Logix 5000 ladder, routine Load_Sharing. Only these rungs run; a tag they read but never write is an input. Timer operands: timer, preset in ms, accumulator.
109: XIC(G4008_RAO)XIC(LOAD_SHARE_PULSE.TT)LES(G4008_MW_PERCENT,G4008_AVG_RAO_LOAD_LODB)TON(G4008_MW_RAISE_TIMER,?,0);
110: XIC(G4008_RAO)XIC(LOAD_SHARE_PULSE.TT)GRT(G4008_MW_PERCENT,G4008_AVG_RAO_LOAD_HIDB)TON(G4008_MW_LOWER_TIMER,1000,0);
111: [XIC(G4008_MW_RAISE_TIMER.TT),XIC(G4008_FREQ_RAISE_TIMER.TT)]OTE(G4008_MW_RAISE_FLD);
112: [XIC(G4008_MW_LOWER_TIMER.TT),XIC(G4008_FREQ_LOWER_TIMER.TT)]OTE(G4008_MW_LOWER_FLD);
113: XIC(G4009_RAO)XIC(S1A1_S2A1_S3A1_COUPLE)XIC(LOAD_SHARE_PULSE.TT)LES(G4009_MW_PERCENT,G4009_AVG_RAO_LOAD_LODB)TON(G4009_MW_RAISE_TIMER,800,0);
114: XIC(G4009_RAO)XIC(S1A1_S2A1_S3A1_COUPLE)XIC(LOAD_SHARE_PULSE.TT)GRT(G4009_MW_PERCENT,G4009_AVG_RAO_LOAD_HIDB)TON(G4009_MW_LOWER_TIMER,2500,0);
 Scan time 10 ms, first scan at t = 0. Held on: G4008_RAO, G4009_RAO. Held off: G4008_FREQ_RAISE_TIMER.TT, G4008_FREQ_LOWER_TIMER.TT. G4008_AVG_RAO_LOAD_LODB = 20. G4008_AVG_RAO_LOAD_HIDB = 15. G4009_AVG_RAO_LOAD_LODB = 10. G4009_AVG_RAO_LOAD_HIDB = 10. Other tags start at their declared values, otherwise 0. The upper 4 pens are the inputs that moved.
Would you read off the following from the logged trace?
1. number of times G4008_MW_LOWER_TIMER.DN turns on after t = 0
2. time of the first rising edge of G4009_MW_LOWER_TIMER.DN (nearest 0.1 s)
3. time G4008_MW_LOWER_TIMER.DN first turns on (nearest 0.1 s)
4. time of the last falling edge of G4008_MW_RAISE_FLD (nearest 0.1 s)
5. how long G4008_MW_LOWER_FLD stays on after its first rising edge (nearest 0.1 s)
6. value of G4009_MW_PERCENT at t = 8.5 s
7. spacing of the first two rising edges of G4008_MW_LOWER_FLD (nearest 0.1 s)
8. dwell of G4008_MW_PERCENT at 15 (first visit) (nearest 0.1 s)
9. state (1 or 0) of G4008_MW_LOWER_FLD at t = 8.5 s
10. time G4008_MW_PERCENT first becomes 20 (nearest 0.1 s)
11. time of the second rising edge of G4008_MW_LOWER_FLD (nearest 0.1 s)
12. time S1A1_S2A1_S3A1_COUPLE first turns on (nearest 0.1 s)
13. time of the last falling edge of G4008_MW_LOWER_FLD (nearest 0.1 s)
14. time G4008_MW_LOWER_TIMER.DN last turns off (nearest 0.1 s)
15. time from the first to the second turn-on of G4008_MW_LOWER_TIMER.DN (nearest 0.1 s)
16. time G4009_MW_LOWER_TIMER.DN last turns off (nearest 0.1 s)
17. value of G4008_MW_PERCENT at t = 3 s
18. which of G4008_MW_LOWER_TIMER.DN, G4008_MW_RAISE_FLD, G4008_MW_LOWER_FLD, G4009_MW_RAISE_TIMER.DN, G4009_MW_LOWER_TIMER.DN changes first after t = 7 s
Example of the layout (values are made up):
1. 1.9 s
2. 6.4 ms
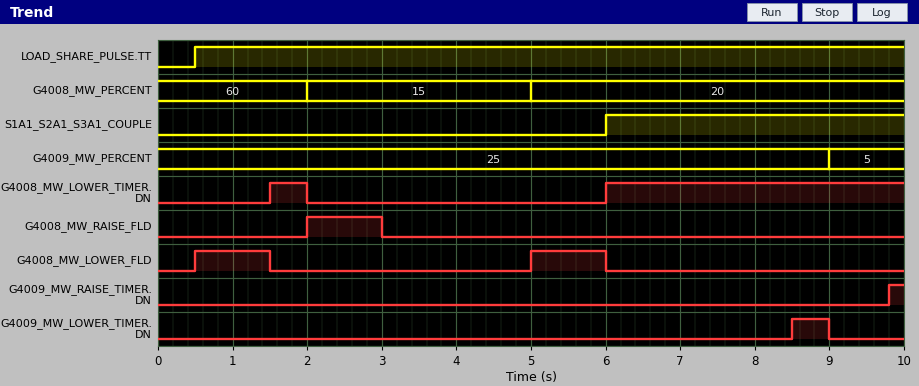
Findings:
1. 2
2. 8.5 s
3. 1.5 s
4. 3.0 s
5. 1.0 s
6. 25
7. 4.5 s
8. 3.0 s
9. 0
10. 5.0 s
11. 5.0 s
12. 6.0 s
13. 6.0 s
14. 2.0 s
15. 4.5 s
16. 9.0 s
17. 15
18. G4009_MW_LOWER_TIMER.DN
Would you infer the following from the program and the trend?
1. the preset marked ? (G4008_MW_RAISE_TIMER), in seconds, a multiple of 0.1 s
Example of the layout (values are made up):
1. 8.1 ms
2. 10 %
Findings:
1. 1.0 s
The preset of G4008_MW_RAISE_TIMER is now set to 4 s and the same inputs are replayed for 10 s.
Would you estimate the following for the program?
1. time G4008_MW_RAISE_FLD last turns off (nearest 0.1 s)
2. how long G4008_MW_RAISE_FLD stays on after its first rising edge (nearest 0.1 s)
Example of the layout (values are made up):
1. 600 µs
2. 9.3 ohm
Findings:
1. 5.0 s
2. 3.0 s
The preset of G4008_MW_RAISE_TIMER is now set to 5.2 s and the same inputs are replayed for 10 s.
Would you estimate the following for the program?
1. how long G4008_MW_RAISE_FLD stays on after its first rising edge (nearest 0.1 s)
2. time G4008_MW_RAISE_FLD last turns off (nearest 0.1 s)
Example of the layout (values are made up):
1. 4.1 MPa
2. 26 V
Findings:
1. 3.0 s
2. 5.0 s
